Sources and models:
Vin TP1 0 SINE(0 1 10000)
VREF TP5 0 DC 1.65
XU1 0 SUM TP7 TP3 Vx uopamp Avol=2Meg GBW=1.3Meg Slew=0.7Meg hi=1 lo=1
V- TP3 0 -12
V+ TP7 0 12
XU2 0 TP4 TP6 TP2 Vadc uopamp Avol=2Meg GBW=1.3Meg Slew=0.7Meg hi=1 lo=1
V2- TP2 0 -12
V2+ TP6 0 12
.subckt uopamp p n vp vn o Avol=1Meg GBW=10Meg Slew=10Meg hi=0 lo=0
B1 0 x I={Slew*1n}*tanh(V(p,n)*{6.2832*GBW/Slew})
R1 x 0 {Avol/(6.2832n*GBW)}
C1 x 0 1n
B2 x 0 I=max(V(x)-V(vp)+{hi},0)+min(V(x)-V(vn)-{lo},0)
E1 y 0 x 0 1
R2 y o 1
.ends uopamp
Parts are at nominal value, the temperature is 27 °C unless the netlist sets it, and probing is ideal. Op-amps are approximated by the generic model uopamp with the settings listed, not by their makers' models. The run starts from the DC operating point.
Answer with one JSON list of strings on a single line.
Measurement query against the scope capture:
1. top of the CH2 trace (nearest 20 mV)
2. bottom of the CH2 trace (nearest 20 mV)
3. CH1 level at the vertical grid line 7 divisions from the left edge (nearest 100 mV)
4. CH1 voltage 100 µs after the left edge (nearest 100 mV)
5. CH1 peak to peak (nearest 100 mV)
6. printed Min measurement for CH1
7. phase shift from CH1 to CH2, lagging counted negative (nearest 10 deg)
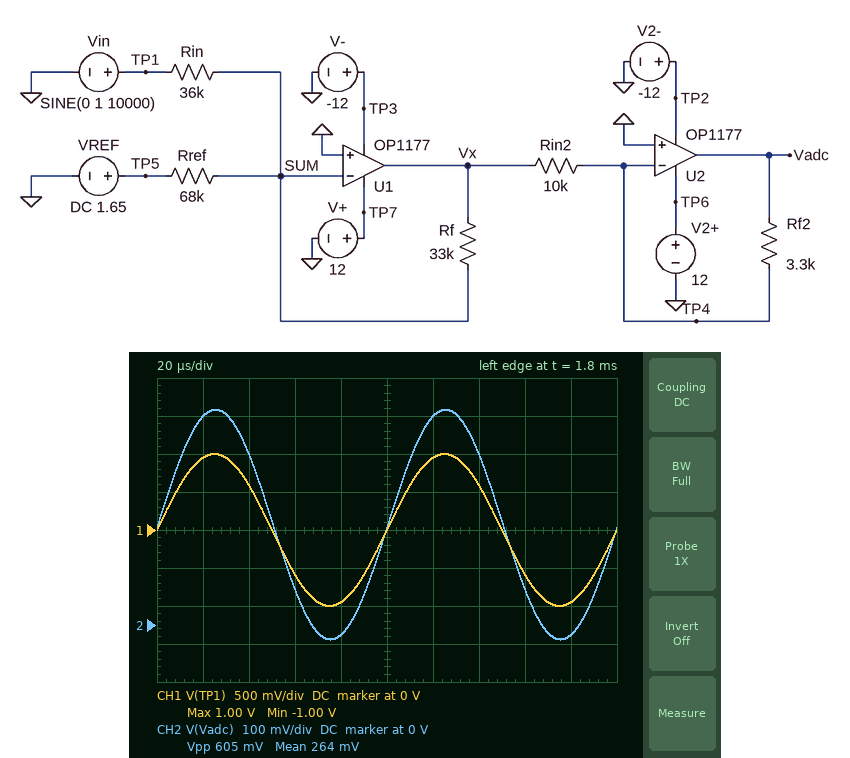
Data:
["560 mV", "-40 mV", "600 mV", "0 V", "2.0 V", "-1.00 V", "0 deg"]
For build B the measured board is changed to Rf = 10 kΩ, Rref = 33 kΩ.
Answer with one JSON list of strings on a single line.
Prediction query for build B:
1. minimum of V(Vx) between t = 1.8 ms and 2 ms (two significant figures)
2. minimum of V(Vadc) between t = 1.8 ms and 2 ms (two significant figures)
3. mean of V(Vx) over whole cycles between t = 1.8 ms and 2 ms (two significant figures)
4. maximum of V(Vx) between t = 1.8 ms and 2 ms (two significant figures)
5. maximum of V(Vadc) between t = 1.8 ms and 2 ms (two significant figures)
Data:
["-780 mV", "73 mV", "-500 mV", "-220 mV", "260 mV"]
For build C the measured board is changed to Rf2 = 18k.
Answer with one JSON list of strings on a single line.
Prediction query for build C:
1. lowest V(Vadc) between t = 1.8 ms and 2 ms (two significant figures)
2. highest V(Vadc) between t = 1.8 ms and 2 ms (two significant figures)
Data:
["-210 mV", "3.1 V"]
